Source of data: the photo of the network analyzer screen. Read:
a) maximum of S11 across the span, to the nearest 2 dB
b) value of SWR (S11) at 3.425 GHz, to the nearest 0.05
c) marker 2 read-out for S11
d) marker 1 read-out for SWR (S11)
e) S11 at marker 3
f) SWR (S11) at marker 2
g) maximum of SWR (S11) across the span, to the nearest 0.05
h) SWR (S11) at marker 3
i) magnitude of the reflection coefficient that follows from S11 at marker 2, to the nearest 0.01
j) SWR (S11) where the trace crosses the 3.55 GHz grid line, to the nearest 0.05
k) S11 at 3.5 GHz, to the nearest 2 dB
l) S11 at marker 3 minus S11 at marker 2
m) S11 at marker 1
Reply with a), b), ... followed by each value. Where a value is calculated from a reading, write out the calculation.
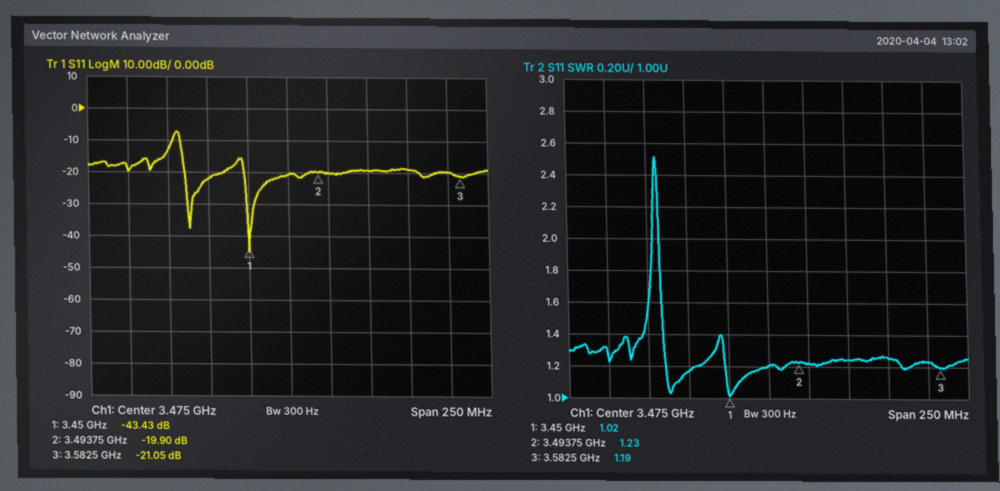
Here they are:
a) -8 dB
b) 1.15
c) -19.90 dB
d) 1.02
e) -21.05 dB
f) 1.23
g) 2.50
h) 1.19
i) 10^(-19.9/20) ≈ 0.10
j) 1.25
k) -20 dB
l) -21.05 − (-19.9) = -1.15 dB
m) -43.43 dB
